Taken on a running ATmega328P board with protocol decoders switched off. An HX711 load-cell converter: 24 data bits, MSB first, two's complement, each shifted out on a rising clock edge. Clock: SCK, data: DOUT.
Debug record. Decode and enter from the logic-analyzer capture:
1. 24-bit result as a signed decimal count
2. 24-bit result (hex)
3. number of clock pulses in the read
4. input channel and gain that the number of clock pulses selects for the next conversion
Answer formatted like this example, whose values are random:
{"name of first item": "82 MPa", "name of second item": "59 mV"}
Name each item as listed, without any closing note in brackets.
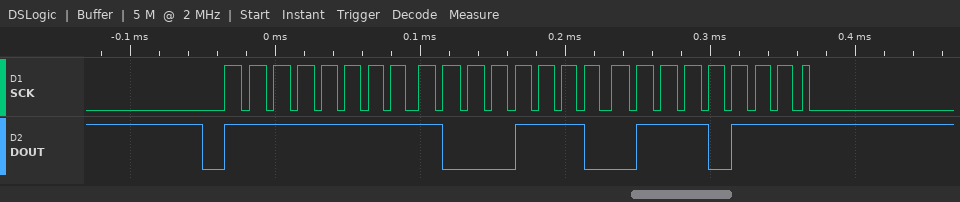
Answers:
{"24-bit result as a signed decimal count": "-29065", "24-bit result": "0xFF8E77", "number of clock pulses in the read": "25", "input channel and gain that the number of clock pulses selects for the next conversion": "channel A, gain 128"}
